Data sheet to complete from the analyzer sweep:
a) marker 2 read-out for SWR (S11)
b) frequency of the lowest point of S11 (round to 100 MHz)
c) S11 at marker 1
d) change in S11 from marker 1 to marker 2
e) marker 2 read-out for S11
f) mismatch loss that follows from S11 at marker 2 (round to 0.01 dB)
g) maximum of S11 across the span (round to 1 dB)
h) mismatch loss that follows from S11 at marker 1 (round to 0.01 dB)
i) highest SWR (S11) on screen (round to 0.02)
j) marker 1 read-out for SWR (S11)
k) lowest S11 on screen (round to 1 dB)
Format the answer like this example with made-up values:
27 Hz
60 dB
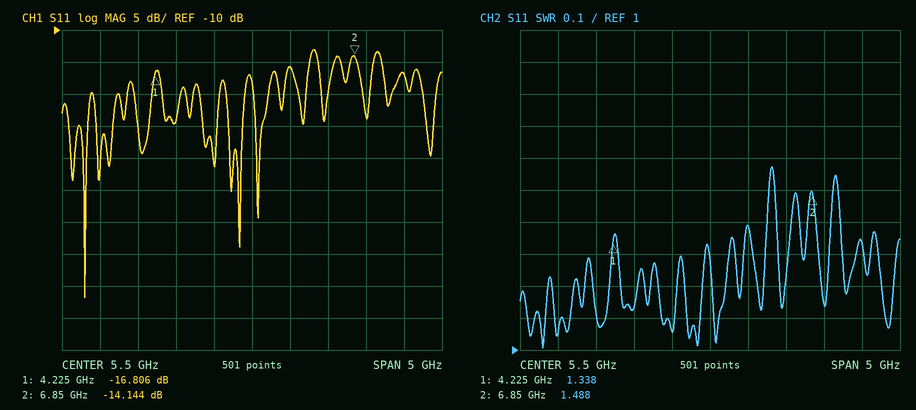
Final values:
1.488
3.3 GHz
-16.806 dB
2.662 dB
-14.144 dB
0.17 dB
-13 dB
0.09 dB
1.58
1.338
-52 dB
